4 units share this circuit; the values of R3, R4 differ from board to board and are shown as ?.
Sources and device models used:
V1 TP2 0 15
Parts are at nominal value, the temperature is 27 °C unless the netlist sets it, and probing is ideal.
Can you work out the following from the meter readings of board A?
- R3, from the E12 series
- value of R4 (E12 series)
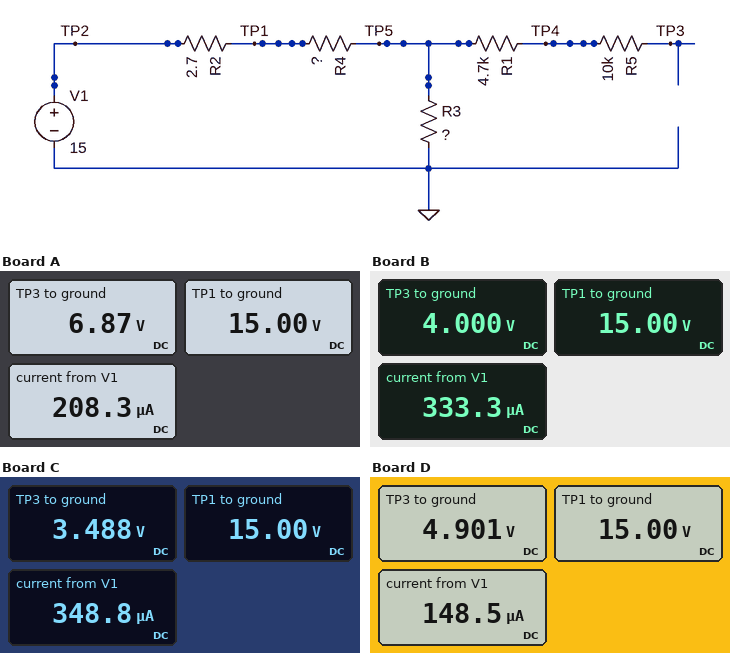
33 kΩ
39 kΩ
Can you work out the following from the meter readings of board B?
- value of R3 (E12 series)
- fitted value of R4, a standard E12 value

12 kΩ
33 kΩ
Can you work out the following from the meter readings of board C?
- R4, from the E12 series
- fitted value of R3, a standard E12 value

33 kΩ
10 kΩ
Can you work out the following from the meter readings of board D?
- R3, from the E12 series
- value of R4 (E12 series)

33 kΩ
68 kΩ
